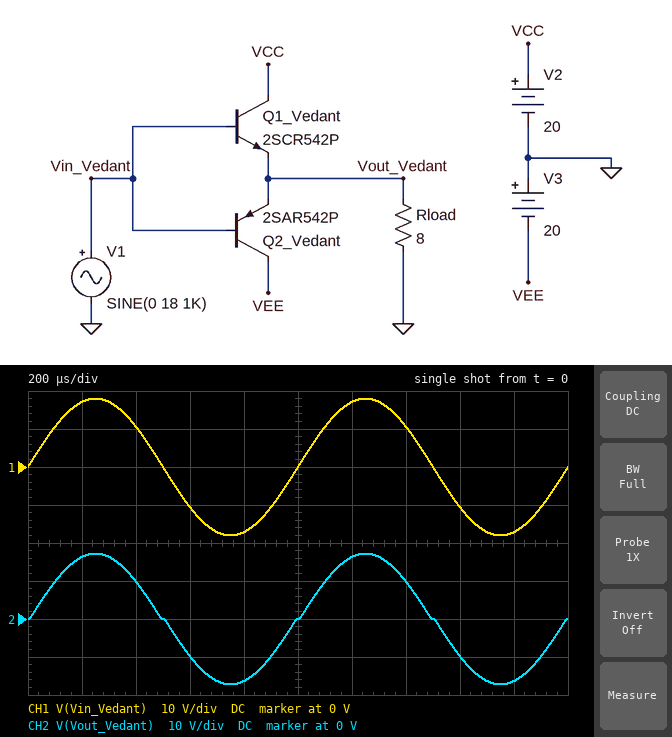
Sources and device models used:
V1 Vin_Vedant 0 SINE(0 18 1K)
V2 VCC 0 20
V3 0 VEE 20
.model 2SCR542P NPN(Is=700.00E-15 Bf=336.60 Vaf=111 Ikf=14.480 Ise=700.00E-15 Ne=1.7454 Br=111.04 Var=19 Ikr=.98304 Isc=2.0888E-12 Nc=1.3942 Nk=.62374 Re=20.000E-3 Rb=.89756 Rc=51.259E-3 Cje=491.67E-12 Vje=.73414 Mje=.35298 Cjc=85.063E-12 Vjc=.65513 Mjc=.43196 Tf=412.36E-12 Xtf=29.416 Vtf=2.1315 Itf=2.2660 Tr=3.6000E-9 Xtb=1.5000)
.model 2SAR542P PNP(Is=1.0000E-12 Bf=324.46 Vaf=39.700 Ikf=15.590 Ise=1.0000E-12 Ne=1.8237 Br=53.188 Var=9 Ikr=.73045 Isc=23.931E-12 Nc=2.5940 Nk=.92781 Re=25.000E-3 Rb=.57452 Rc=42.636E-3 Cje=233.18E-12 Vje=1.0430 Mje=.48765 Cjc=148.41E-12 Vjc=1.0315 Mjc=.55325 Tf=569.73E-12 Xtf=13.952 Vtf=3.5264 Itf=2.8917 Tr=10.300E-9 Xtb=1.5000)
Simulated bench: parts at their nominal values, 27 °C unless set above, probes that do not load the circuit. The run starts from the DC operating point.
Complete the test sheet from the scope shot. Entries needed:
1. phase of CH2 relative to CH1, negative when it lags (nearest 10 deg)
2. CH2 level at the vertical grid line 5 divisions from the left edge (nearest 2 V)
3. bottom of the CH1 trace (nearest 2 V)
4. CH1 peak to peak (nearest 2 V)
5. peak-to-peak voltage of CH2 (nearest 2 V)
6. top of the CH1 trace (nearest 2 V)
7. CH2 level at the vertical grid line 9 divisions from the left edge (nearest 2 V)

0 deg
0 V
-18 V
36 V
34 V
18 V
-16 V
